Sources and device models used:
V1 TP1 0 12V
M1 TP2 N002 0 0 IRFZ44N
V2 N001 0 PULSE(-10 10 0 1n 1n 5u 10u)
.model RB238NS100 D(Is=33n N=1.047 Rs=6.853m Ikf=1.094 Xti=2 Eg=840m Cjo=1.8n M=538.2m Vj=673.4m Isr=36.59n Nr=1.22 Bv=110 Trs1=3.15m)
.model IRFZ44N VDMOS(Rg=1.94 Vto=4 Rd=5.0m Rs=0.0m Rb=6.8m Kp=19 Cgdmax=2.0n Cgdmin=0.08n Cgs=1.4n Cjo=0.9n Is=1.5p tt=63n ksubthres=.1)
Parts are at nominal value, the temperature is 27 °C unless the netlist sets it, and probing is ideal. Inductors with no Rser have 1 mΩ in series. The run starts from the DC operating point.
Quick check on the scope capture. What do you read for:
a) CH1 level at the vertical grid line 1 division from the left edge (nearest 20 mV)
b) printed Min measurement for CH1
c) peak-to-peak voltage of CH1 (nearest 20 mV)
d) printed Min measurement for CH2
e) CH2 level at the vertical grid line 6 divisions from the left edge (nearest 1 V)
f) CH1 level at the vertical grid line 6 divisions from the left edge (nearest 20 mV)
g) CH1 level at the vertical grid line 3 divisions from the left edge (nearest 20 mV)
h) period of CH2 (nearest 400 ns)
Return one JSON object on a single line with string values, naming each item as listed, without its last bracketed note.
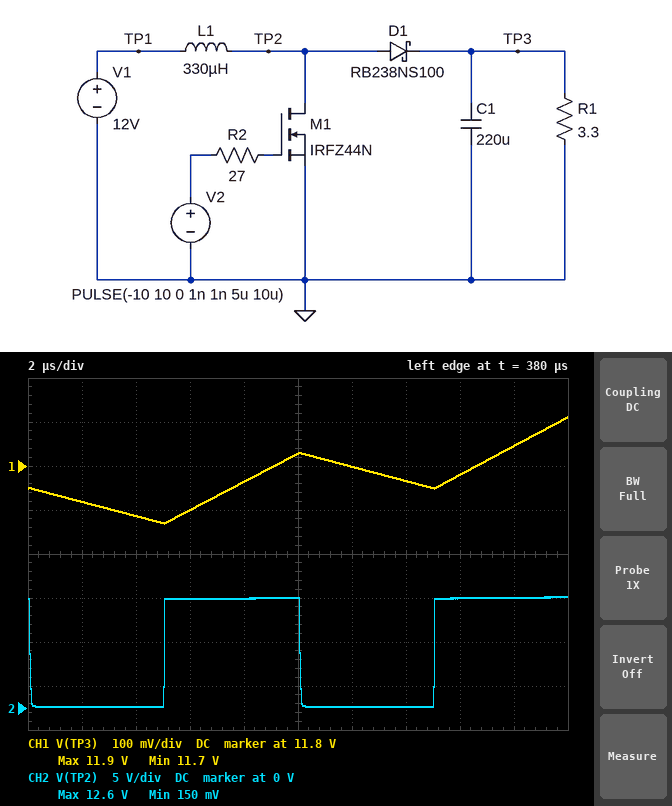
{"CH1 level at the vertical grid line 1 division from the left edge": "11.72 V", "printed Min measurement for CH1": "11.7 V", "peak-to-peak voltage of CH1": "240 mV", "printed Min measurement for CH2": "150 mV", "CH2 level at the vertical grid line 6 divisions from the left edge": "0 V", "CH1 level at the vertical grid line 6 divisions from the left edge": "11.80 V", "CH1 level at the vertical grid line 3 divisions from the left edge": "11.70 V", "period of CH2": "10.0 µs"}
